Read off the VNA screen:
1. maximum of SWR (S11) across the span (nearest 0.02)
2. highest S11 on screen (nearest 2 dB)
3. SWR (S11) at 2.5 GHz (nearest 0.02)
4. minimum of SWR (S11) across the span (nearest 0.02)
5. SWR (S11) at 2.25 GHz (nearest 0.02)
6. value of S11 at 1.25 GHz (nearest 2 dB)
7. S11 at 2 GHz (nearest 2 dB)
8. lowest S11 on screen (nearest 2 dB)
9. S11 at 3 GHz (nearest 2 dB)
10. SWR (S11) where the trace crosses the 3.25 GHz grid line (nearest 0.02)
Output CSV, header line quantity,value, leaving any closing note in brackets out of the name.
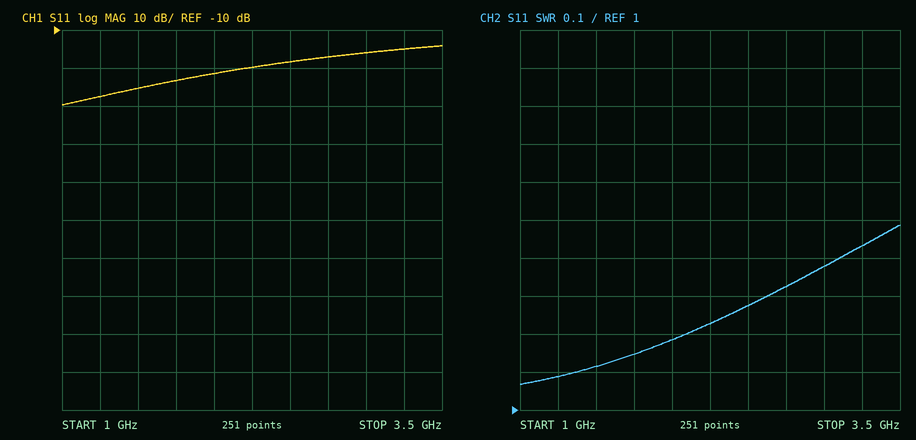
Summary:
quantity,value
maximum of SWR (S11) across the span,1.48
highest S11 on screen,-14 dB
SWR (S11) at 2.5 GHz,1.28
minimum of SWR (S11) across the span,1.06
SWR (S11) at 2.25 GHz,1.22
value of S11 at 1.25 GHz,-28 dB
S11 at 2 GHz,-22 dB
lowest S11 on screen,-30 dB
S11 at 3 GHz,-16 dB
SWR (S11) where the trace crosses the 3.25 GHz grid line,1.44
